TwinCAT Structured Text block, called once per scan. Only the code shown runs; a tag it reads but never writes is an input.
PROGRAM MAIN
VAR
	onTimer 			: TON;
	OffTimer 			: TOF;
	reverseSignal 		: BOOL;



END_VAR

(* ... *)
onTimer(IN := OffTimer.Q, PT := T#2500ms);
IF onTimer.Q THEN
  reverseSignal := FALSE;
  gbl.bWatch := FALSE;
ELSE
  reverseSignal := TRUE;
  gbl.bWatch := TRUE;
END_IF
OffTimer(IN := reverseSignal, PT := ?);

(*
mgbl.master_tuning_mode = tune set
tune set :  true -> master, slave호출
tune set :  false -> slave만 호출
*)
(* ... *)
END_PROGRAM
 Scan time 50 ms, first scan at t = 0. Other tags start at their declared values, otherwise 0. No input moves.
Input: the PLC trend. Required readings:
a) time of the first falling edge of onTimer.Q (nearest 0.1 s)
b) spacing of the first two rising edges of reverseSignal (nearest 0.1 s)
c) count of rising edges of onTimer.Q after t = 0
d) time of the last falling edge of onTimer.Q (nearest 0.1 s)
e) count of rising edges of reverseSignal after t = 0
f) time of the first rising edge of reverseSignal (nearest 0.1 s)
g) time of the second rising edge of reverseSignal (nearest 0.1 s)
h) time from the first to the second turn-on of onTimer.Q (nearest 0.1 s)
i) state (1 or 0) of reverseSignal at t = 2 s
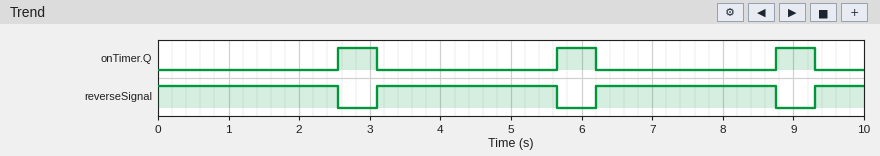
3.1 s
3.1 s
3
9.3 s
3
3.1 s
6.2 s
3.1 s
1
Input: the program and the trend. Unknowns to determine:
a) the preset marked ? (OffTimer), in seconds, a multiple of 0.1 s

0.5 s
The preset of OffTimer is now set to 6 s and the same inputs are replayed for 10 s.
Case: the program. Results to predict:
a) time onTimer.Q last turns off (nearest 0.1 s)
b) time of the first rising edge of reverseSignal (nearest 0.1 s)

8.6 s
8.6 s
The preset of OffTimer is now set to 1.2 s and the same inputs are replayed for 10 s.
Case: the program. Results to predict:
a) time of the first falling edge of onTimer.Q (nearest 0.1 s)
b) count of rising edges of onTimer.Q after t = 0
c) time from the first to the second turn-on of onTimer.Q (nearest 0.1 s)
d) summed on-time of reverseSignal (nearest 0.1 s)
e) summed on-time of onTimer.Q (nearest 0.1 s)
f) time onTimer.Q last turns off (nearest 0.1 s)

3.8 s
2
3.8 s
7.5 s
2.5 s
7.6 s
